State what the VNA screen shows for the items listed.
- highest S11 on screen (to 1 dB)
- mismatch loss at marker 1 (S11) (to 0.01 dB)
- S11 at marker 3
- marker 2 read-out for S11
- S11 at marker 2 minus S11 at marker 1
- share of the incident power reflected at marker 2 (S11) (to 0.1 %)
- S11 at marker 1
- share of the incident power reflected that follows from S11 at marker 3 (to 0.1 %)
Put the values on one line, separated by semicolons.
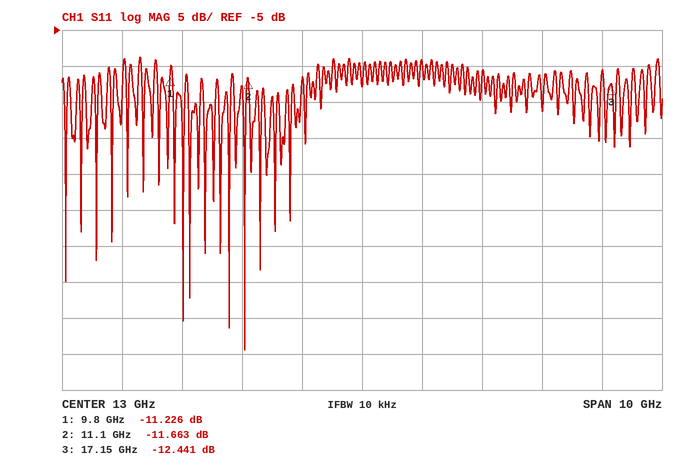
-9 dB; 0.34 dB; -12.441 dB; -11.663 dB; -0.437 dB; 6.8 %; -11.226 dB; 5.7 %
